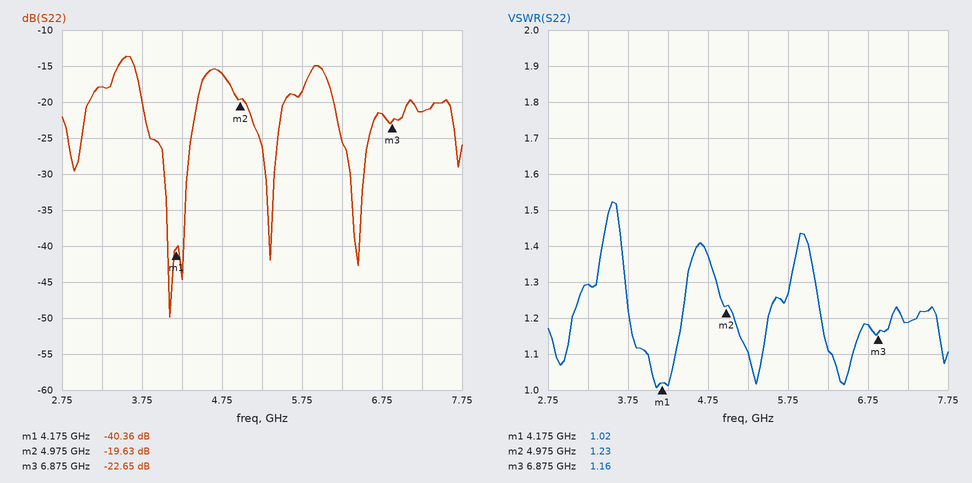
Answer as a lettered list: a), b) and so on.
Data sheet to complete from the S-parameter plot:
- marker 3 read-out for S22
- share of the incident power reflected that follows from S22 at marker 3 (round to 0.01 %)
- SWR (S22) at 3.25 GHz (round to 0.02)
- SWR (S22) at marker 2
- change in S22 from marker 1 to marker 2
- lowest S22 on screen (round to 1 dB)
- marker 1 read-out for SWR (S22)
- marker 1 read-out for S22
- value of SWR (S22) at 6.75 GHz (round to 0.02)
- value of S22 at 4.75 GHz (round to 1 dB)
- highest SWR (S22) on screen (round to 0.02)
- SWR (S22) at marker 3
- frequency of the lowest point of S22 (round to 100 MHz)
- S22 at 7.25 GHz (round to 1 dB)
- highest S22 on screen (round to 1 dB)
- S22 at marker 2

a) -22.65 dB
b) 0.54 %
c) 1.30
d) 1.23
e) 20.73 dB
f) -50 dB
g) 1.02
h) -40.36 dB
i) 1.18
j) -16 dB
k) 1.52
l) 1.16
m) 4.1 GHz
n) -21 dB
o) -14 dB
p) -19.63 dB
